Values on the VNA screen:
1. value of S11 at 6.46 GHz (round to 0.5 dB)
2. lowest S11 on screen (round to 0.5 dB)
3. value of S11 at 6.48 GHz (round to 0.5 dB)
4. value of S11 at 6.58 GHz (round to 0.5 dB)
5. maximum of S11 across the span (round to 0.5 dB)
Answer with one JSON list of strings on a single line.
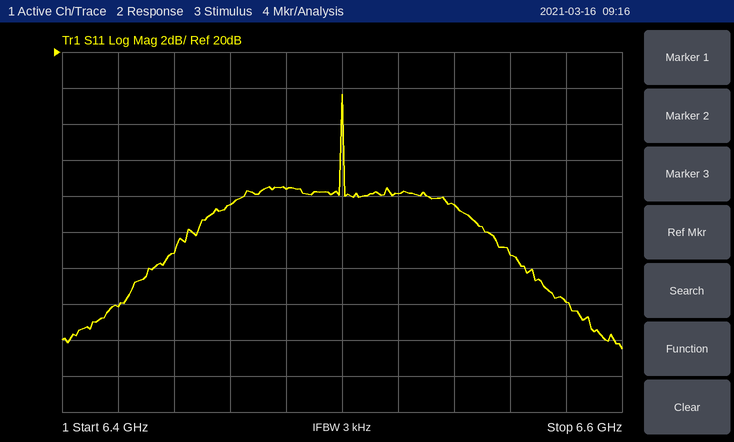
["11.5 dB", "3.5 dB", "12.5 dB", "6.0 dB", "17.5 dB"]
